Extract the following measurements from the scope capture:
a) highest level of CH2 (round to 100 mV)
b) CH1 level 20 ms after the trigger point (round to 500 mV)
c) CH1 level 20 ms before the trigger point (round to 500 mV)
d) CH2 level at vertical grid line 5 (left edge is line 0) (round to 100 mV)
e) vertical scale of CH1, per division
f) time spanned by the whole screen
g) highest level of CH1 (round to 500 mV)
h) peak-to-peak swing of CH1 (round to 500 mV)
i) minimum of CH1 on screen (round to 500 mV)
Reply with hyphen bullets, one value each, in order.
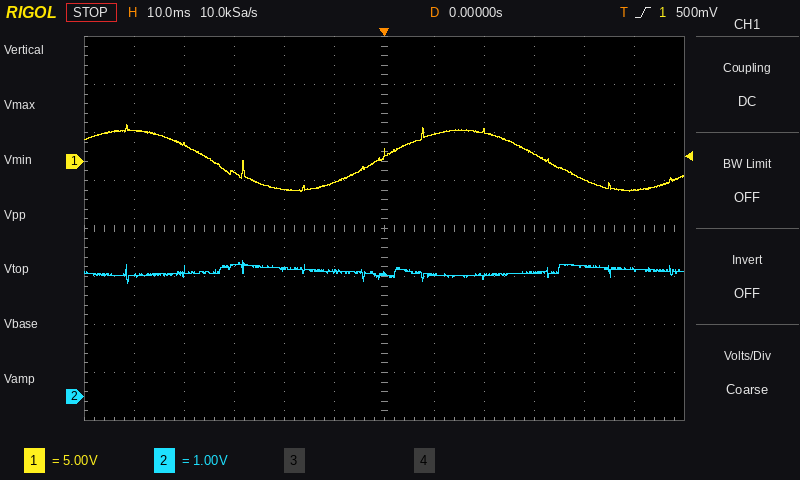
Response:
- 2.8 V
- 3.0 V
- -3.0 V
- 2.6 V
- 5 V
- 120 ms
- 4.0 V
- 7.0 V
- -3.0 V
